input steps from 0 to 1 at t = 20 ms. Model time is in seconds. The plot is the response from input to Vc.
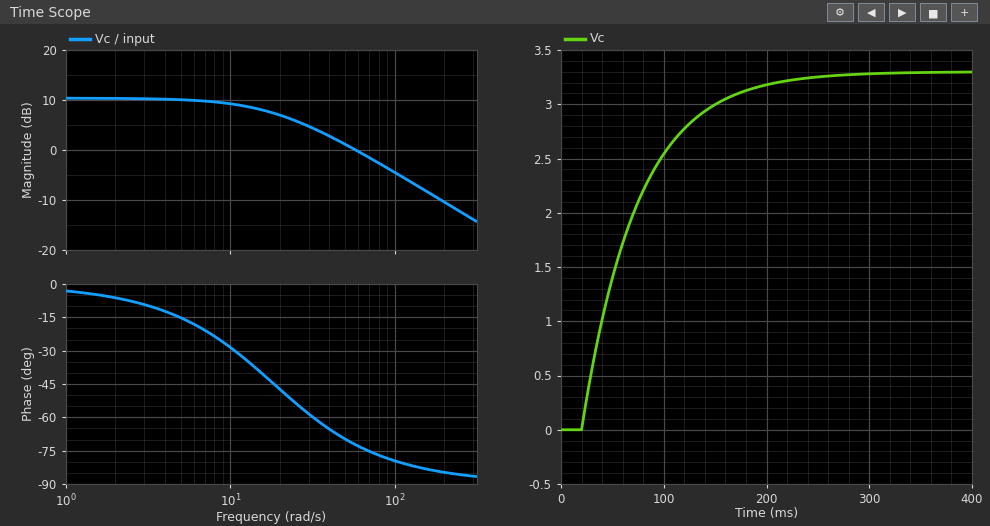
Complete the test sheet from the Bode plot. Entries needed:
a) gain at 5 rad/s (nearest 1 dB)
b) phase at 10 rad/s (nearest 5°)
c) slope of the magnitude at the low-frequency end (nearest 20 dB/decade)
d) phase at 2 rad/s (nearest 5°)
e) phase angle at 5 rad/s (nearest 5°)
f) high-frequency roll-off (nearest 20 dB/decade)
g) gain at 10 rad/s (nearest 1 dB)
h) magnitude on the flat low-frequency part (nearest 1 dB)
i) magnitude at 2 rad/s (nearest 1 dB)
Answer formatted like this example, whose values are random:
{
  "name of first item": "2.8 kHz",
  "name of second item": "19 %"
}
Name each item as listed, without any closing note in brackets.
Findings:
{
  "gain at 5 rad/s": "10 dB",
  "phase at 10 rad/s": "-30°",
  "slope of the magnitude at the low-frequency end": "0 dB/decade",
  "phase at 2 rad/s": "-5°",
  "phase angle at 5 rad/s": "-15°",
  "high-frequency roll-off": "-20 dB/decade",
  "gain at 10 rad/s": "9 dB",
  "magnitude on the flat low-frequency part": "10 dB",
  "magnitude at 2 rad/s": "10 dB"
}
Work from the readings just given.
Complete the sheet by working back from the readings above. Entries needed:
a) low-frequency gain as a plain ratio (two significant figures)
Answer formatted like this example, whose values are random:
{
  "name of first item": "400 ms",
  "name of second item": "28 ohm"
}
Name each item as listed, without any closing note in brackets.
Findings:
{
  "low-frequency gain as a plain ratio": "3.2"
}
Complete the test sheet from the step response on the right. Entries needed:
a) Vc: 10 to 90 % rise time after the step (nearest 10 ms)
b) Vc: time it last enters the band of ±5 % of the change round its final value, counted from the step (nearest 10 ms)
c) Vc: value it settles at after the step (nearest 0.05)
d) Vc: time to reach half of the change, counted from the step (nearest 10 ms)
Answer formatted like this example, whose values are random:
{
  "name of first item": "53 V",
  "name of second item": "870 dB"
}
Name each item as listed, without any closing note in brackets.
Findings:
{
  "Vc: 10 to 90 % rise time after the step": "120 ms",
  "Vc: time it last enters the band of ±5 % of the change round its final value, counted from the step": "160 ms",
  "Vc: value it settles at after the step": "3.30",
  "Vc: time to reach half of the change, counted from the step": "40 ms"
}
